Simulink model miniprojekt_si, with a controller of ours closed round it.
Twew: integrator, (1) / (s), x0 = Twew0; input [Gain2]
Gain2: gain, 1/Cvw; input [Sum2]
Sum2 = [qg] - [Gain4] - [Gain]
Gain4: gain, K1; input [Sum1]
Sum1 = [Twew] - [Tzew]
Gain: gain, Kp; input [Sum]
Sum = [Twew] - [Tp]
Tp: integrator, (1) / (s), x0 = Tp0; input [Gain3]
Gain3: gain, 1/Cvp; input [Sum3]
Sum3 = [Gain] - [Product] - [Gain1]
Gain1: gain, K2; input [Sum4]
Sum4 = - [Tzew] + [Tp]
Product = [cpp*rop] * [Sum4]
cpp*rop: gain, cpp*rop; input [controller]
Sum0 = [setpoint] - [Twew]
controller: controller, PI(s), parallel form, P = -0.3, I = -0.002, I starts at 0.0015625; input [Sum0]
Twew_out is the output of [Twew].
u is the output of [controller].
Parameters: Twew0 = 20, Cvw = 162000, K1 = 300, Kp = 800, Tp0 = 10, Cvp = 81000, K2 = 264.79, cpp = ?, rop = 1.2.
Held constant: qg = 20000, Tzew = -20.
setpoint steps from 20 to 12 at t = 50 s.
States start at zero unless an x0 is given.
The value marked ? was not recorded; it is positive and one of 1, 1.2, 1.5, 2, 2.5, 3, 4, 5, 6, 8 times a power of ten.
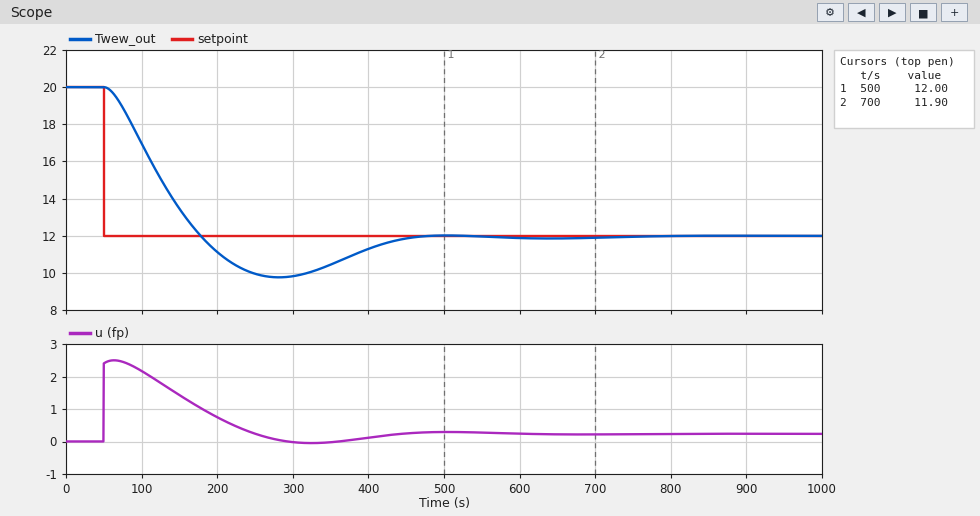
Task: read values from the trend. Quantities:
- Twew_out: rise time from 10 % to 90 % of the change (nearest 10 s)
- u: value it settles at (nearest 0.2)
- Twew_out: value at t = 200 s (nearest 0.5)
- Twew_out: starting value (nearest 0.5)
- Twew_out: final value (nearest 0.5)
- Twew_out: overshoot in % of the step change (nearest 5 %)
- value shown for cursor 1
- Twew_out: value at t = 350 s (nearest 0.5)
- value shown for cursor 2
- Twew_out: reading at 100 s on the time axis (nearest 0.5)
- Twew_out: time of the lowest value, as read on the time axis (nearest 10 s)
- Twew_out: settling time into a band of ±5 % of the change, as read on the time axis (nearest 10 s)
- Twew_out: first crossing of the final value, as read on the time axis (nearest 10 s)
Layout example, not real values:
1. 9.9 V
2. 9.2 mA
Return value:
1. 90 s
2. 0.2
3. 11.0
4. 20.0
5. 12.0
6. 30 %
7. 12.00
8. 10.5
9. 11.90
10. 17.0
11. 280 s
12. 420 s
13. 180 s
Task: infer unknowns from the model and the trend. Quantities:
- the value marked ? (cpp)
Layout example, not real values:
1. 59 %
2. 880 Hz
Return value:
1. 1000
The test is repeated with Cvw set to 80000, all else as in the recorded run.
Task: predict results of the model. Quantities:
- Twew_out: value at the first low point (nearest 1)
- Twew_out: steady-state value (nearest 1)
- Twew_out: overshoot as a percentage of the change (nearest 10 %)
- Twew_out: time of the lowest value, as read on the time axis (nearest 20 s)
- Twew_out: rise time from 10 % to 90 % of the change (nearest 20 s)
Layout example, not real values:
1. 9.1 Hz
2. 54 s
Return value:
1. 10
2. 12
3. 20 %
4. 180 s
5. 60 s
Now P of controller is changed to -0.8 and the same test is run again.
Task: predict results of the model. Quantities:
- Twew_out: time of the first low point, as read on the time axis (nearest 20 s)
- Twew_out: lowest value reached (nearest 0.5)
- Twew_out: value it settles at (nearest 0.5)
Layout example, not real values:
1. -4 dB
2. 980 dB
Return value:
1. 200 s
2. 10.5
3. 12.0
